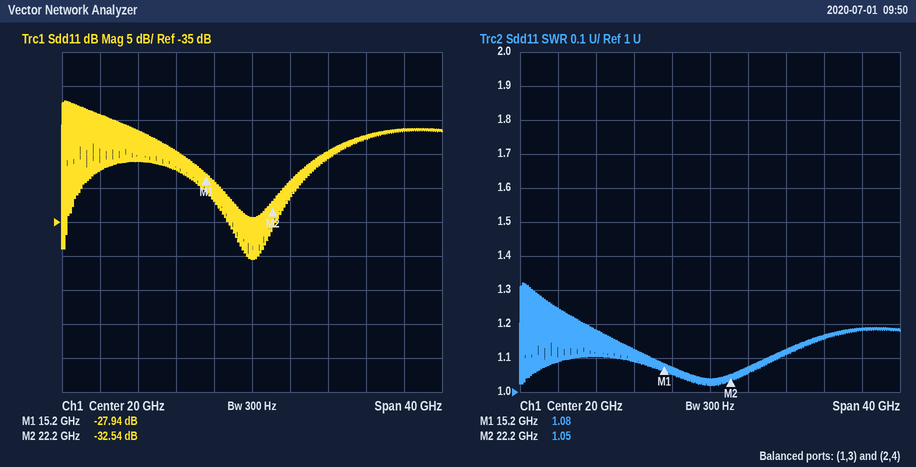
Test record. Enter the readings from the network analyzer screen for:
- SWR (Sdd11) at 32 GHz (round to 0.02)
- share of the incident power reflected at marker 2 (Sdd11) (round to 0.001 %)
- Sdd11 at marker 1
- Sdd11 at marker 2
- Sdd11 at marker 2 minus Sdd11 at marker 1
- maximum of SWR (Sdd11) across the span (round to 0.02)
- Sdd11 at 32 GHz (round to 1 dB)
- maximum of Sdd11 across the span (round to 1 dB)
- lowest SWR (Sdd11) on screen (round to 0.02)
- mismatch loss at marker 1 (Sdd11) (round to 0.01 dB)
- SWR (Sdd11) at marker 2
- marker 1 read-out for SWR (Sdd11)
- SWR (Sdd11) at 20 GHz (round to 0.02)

1.16
0.056 %
-27.94 dB
-32.54 dB
-4.60 dB
1.32
-22 dB
-17 dB
1.02
0.01 dB
1.05
1.08
1.02
